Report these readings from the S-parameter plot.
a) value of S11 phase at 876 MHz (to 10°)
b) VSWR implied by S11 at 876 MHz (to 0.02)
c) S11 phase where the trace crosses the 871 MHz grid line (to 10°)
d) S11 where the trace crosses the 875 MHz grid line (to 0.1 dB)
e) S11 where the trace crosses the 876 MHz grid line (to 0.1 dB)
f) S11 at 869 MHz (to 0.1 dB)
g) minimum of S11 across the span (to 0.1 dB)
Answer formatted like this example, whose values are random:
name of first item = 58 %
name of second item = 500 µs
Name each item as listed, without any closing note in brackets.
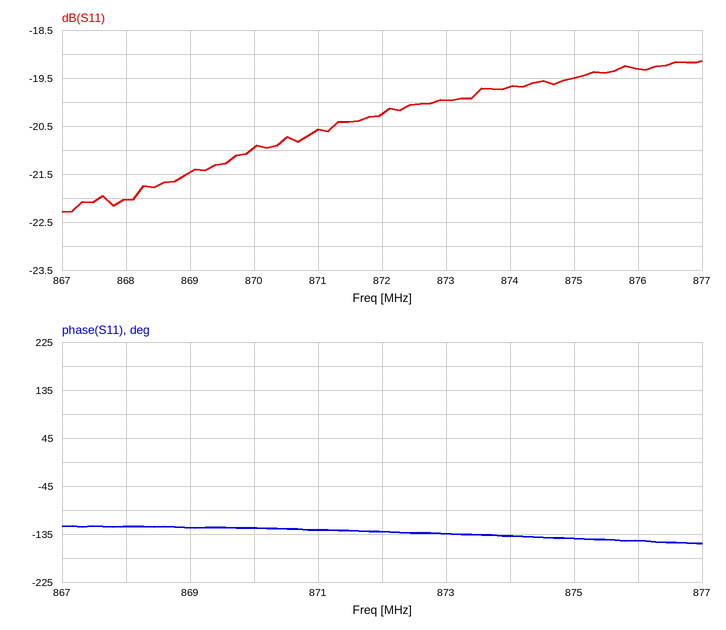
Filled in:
value of S11 phase at 876 MHz = -150°
VSWR implied by S11 at 876 MHz = 1.24
S11 phase where the trace crosses the 871 MHz grid line = -130°
S11 where the trace crosses the 875 MHz grid line = -19.5 dB
S11 where the trace crosses the 876 MHz grid line = -19.3 dB
S11 at 869 MHz = -21.5 dB
minimum of S11 across the span = -22.3 dB
